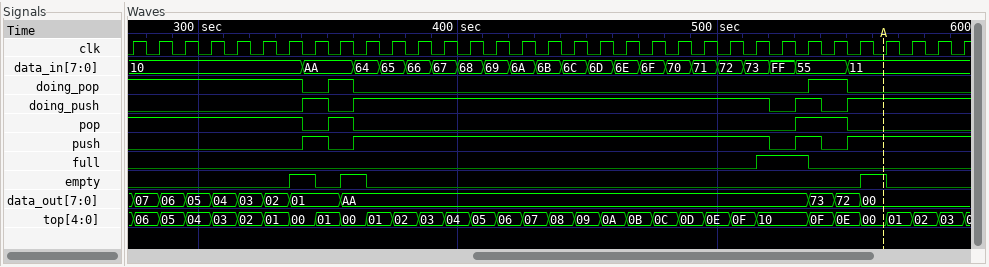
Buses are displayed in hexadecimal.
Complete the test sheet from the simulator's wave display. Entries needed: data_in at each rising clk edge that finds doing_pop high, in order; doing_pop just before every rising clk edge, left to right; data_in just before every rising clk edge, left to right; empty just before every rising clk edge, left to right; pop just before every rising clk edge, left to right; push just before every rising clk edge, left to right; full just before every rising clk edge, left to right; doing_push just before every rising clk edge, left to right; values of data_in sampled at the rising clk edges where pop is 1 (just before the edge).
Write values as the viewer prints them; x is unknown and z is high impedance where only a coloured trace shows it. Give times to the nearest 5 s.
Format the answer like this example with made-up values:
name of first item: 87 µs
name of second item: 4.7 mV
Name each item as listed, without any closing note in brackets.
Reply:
data_in at each rising clk edge that finds doing_pop high, in order: 10, 10, 10, 10, 10, 10, 10, AA, 55
doing_pop just before every rising clk edge, left to right: 1 1 1 1 1 1 1 0 1 0 0 0 0 0 0 0 0 0 0 0 0 0 0 0 0 0 0 1 0 0 0 0 0
data_in just before every rising clk edge, left to right: 10, 10, 10, 10, 10, 10, 10, AA, AA, 64, 65, 66, 67, 68, 69, 6A, 6B, 6C, 6D, 6E, 6F, 70, 71, 72, 73, FF, 55, 55, 11, 11, 11, 11, 11
empty just before every rising clk edge, left to right: 0 0 0 0 0 0 0 1 0 1 0 0 0 0 0 0 0 0 0 0 0 0 0 0 0 0 0 0 0 1 0 0 0
pop just before every rising clk edge, left to right: 1 1 1 1 1 1 1 0 1 0 0 0 0 0 0 0 0 0 0 0 0 0 0 0 0 0 1 1 0 0 0 0 0
push just before every rising clk edge, left to right: 0 0 0 0 0 0 0 1 0 1 1 1 1 1 1 1 1 1 1 1 1 1 1 1 1 0 1 0 1 1 1 1 1
full just before every rising clk edge, left to right: 0 0 0 0 0 0 0 0 0 0 0 0 0 0 0 0 0 0 0 0 0 0 0 0 0 1 1 0 0 0 0 0 0
doing_push just before every rising clk edge, left to right: 0 0 0 0 0 0 0 1 0 1 1 1 1 1 1 1 1 1 1 1 1 1 1 1 1 0 1 0 1 1 1 1 1
values of data_in sampled at the rising clk edges where pop is 1: 10, 10, 10, 10, 10, 10, 10, AA, 55, 55
